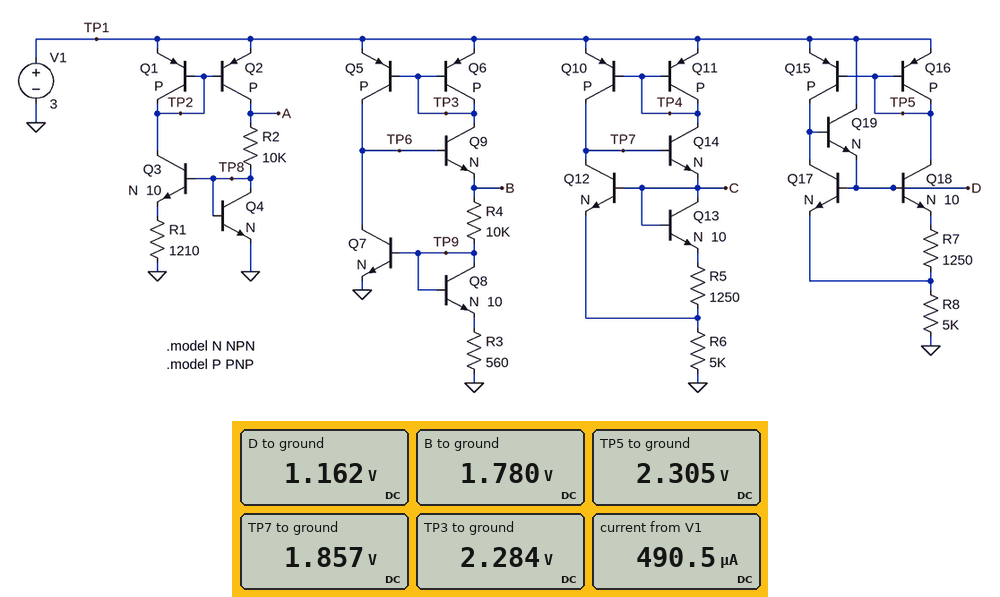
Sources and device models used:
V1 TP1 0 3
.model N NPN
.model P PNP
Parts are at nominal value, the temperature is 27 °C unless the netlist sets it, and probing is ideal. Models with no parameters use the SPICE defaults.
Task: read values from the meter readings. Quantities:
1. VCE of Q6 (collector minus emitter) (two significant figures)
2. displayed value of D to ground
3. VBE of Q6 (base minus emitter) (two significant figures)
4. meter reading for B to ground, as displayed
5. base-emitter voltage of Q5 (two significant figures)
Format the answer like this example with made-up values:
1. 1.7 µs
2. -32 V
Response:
1. -720 mV
2. 1.162 V
3. -720 mV
4. 1.780 V
5. -720 mV
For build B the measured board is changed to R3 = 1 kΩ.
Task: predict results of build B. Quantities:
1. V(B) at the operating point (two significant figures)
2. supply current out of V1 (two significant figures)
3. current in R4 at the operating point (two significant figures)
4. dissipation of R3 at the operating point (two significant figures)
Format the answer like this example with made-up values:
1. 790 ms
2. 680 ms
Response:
1. 1.3 V
2. 400 µA
3. 60 µA
4. 3.5 µW
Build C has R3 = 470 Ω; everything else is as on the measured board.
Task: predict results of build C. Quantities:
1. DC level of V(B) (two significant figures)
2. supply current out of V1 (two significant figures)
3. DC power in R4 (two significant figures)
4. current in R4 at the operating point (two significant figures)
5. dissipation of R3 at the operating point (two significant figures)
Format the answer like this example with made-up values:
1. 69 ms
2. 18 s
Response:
1. 2.0 V
2. 530 µA
3. 160 µW
4. 130 µA
5. 7.4 µW
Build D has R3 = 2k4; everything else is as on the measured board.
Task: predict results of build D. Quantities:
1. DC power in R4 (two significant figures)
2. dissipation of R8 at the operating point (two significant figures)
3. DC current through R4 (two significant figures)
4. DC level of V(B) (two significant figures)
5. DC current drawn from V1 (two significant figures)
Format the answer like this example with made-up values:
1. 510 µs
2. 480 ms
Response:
1. 6.2 µW
2. 44 µW
3. 25 µA
4. 930 mV
5. 330 µA
